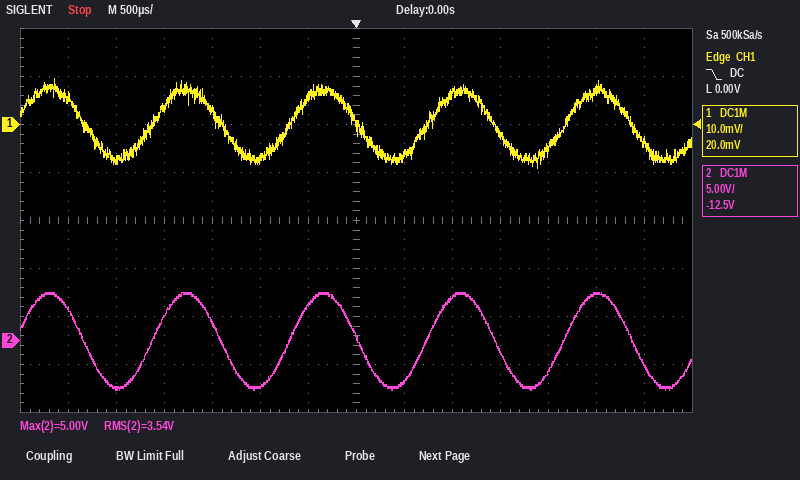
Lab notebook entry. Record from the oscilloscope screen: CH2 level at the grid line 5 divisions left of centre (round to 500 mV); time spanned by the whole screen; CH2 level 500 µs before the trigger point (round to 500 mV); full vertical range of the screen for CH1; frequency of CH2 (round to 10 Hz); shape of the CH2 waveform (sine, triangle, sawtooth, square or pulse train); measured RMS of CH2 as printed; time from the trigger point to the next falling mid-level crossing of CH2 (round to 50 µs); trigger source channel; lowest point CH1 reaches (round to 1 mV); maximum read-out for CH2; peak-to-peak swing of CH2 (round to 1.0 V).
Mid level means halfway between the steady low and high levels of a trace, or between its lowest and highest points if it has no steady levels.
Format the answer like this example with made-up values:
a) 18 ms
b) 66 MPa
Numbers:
a) -5.0 V
b) 7 ms
c) 3.5 V
d) 80 mV
e) 700 Hz
f) sine
g) 3.54 V
h) 1.45 ms
i) CH1
j) -9 mV
k) 5.00 V
l) 10.0 V
